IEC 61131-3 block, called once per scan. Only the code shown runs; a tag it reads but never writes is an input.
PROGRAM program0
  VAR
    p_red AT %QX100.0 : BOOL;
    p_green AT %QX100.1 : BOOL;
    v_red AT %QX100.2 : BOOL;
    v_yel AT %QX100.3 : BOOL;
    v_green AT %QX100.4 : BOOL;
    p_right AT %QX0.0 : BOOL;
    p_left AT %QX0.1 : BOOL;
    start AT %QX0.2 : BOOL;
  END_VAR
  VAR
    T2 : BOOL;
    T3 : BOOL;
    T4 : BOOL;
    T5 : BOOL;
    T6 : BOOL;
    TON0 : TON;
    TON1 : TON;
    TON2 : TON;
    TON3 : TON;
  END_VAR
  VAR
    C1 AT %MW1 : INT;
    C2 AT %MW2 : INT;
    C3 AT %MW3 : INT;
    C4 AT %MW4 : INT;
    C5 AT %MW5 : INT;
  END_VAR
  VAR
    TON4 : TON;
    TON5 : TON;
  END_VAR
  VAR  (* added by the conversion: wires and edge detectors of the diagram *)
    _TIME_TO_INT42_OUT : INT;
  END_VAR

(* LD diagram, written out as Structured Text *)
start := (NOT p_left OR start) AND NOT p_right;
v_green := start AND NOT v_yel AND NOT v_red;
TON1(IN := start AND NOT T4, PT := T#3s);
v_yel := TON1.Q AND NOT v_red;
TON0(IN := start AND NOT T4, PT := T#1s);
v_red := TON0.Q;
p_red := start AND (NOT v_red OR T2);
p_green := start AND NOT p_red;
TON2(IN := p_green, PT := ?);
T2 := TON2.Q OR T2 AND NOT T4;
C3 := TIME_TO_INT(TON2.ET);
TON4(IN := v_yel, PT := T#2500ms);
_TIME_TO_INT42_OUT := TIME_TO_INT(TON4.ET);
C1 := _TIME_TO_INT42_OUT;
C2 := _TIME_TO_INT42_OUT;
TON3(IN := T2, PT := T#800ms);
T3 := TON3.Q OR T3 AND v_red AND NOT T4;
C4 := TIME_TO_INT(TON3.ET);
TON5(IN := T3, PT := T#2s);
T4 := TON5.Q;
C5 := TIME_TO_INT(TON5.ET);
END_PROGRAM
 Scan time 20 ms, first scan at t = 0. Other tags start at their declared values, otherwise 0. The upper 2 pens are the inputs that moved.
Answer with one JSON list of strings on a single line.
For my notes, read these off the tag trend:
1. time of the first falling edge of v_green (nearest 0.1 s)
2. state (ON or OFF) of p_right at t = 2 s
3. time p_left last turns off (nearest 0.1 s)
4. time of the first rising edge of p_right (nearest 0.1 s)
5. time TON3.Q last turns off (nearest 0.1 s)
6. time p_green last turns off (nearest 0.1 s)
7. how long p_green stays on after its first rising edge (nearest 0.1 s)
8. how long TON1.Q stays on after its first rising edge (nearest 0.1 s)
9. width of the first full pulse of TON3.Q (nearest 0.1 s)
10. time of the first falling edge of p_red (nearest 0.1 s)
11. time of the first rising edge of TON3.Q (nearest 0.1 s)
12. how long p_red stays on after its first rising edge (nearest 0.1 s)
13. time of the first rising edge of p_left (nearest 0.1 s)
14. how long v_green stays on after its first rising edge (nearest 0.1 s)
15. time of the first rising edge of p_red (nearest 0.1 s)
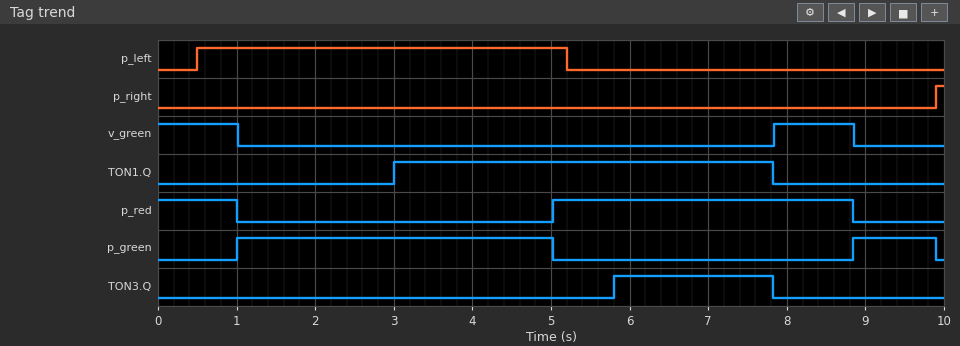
["1.0 s", "OFF", "5.2 s", "9.9 s", "7.8 s", "9.9 s", "4.0 s", "4.8 s", "2.0 s", "1.0 s", "5.8 s", "3.8 s", "0.5 s", "1.0 s", "5.0 s"]
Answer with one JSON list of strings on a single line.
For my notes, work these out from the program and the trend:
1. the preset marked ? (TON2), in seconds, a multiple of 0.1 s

["4.0 s"]
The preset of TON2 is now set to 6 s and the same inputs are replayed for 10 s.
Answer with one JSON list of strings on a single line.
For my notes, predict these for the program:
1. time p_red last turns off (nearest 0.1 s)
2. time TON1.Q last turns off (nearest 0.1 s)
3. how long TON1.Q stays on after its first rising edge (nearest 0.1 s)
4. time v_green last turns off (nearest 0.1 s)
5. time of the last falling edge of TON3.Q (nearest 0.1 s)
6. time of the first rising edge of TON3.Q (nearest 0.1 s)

["9.9 s", "9.8 s", "6.8 s", "9.9 s", "9.8 s", "7.8 s"]
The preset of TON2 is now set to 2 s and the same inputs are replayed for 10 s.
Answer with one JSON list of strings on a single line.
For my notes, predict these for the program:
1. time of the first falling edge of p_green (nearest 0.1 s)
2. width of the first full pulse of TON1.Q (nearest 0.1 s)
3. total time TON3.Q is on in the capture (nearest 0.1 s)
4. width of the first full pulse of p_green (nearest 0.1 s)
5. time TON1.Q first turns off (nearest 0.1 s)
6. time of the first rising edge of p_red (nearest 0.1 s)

["3.0 s", "2.8 s", "2.4 s", "2.0 s", "5.8 s", "3.0 s"]
